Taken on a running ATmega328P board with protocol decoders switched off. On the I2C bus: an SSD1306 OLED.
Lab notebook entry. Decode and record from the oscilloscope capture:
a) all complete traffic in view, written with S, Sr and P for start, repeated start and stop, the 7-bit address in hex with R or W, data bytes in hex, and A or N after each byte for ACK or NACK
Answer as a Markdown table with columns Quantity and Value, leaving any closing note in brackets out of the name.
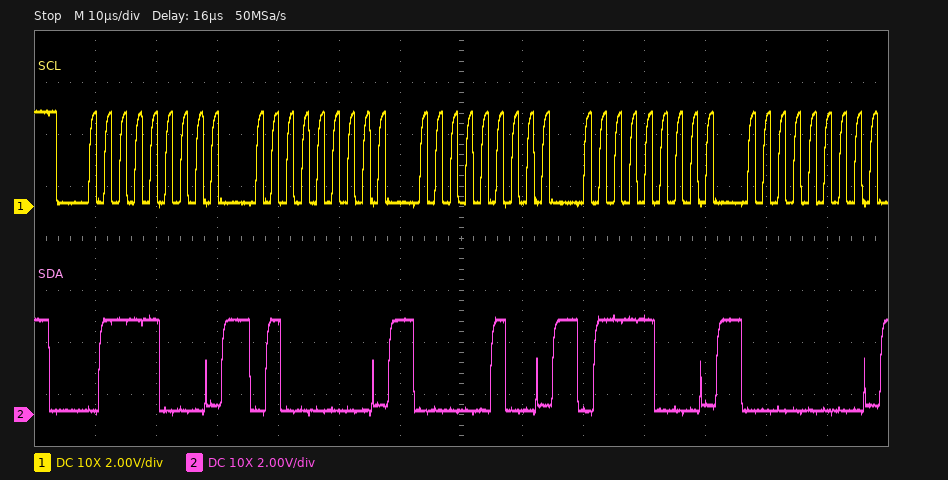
| Quantity | Value |
|---|---|
| all complete traffic in view, written with S, Sr and P for start, repeated start and stop, the 7-bit address in hex with R or W, data bytes in hex, and A or N after each byte for ACK or NACK | S 3CW A 40 A 04 A 78 A 00 A |
